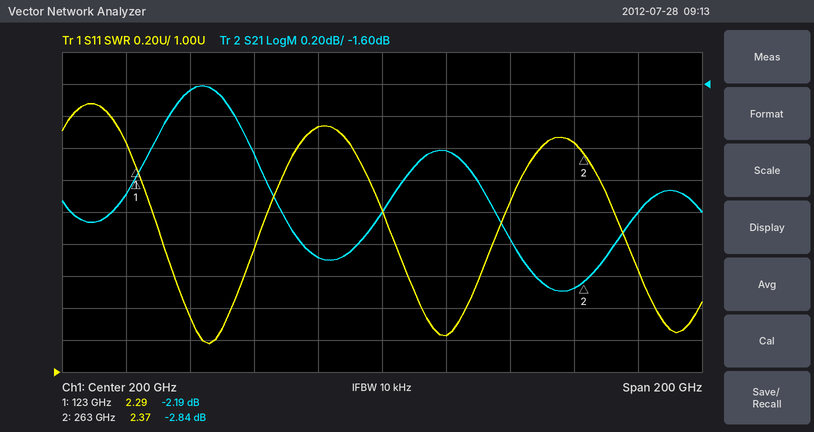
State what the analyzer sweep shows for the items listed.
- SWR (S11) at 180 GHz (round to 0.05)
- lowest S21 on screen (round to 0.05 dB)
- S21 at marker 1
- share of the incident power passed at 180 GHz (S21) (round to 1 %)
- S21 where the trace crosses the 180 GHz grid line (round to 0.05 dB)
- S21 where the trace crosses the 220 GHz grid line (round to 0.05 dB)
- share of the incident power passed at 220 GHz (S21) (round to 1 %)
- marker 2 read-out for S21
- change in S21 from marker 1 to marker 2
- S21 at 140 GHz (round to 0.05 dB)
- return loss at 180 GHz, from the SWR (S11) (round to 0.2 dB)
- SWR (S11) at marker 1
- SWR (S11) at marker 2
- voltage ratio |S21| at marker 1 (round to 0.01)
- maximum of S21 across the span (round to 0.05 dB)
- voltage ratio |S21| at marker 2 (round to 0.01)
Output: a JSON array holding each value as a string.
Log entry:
["2.55", "-2.90 dB", "-2.19 dB", "54 %", "-2.70 dB", "-2.00 dB", "63 %", "-2.84 dB", "-0.65 dB", "-1.65 dB", "7.2 dB", "2.29", "2.37", "0.78", "-1.60 dB", "0.72"]
